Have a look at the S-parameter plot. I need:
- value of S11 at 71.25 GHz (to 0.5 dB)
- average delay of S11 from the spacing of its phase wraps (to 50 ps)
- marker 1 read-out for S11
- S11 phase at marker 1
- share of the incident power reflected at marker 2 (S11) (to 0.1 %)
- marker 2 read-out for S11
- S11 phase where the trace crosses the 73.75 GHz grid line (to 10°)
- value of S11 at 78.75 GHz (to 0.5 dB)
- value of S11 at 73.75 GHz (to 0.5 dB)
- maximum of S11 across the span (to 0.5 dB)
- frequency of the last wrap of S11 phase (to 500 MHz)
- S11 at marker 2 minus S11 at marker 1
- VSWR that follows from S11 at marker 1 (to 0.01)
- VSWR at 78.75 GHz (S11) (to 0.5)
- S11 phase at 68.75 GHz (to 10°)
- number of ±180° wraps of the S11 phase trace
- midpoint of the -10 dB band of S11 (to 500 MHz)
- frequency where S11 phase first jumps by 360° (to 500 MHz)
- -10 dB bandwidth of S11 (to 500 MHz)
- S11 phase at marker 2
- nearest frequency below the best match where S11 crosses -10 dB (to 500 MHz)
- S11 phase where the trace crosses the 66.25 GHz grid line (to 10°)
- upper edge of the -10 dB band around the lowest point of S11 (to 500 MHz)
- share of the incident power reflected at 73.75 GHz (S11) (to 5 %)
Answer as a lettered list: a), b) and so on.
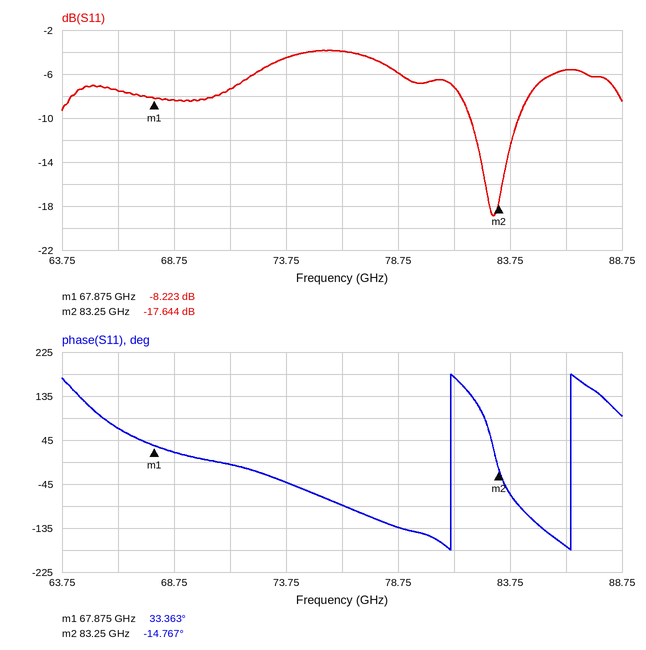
a) -7.5 dB
b) 200 ps
c) -8.223 dB
d) 33.363°
e) 1.7 %
f) -17.644 dB
g) -40°
h) -6.0 dB
i) -4.5 dB
j) -4.0 dB
k) 86.5 GHz
l) -9.421 dB
m) 2.27
n) 3.0
o) 20°
p) 2
q) 83.0 GHz
r) 81.0 GHz
s) 2.0 GHz
t) -14.767°
u) 82.0 GHz
v) 70°
w) 84.0 GHz
x) 35 %
